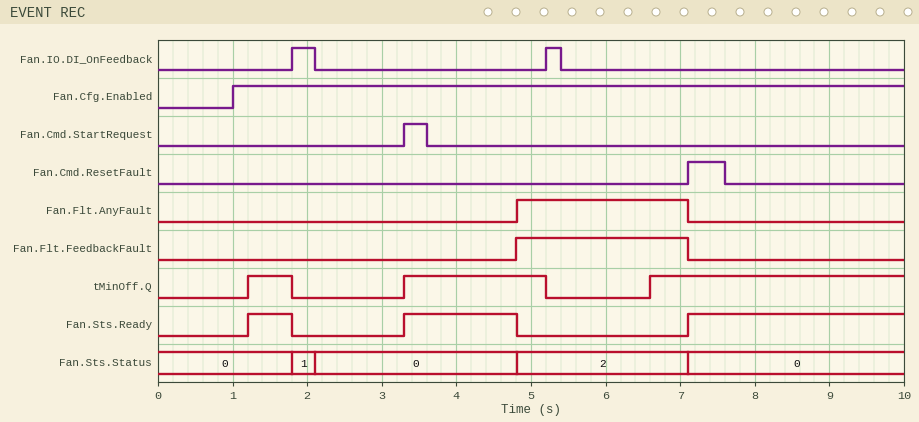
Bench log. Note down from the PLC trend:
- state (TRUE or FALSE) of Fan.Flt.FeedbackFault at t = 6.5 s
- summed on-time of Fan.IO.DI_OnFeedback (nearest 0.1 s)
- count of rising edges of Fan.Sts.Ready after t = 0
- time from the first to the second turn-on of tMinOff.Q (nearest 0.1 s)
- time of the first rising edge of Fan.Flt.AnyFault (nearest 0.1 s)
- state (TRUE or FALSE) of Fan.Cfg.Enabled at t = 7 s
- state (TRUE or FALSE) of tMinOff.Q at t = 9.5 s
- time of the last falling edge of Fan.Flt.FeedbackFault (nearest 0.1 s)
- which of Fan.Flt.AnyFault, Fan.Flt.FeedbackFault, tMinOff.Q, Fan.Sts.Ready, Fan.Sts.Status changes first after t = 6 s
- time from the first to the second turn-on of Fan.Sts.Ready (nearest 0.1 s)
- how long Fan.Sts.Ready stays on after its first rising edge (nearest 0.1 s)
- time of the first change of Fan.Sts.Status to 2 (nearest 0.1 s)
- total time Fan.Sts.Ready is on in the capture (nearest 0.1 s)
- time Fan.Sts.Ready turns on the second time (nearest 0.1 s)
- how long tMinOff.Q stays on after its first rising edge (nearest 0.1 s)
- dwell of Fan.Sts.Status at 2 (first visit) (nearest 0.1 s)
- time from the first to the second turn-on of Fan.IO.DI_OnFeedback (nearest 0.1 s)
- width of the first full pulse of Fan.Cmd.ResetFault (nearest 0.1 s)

TRUE
0.5 s
3
2.1 s
4.8 s
TRUE
TRUE
7.1 s
tMinOff.Q
2.1 s
0.6 s
4.8 s
5.0 s
3.3 s
0.6 s
2.3 s
3.4 s
0.5 s
